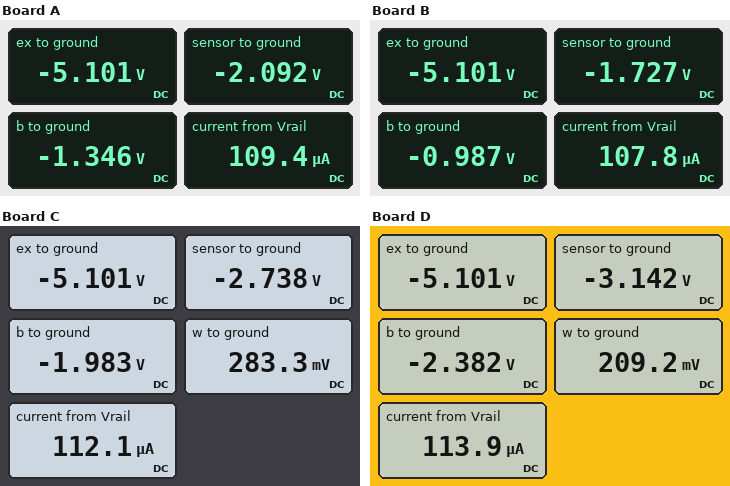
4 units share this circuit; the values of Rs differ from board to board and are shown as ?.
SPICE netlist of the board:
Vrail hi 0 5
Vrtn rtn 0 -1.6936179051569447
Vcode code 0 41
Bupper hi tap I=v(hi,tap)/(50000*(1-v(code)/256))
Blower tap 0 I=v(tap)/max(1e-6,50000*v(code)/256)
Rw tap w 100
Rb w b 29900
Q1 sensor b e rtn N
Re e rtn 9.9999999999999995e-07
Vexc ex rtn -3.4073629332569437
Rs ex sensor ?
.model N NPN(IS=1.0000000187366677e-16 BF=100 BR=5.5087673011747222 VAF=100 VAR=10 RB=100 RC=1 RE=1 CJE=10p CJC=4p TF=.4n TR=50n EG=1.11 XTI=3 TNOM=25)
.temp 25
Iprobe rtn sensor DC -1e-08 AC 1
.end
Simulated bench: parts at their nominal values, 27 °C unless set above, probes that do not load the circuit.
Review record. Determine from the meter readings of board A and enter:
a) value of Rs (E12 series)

8.2 kΩ
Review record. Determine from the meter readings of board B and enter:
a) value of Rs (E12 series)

15 kΩ
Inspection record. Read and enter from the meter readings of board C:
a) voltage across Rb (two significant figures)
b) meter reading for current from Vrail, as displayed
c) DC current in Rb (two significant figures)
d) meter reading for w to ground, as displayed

2.3 V
112.1 µA
76 µA
283.3 mV
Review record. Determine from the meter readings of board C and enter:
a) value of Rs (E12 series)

4.7 kΩ
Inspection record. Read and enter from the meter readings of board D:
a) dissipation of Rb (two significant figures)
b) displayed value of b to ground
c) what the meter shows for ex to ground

220 µW
-2.382 V
-5.101 V
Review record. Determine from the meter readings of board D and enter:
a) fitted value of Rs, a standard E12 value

3.3 kΩ
